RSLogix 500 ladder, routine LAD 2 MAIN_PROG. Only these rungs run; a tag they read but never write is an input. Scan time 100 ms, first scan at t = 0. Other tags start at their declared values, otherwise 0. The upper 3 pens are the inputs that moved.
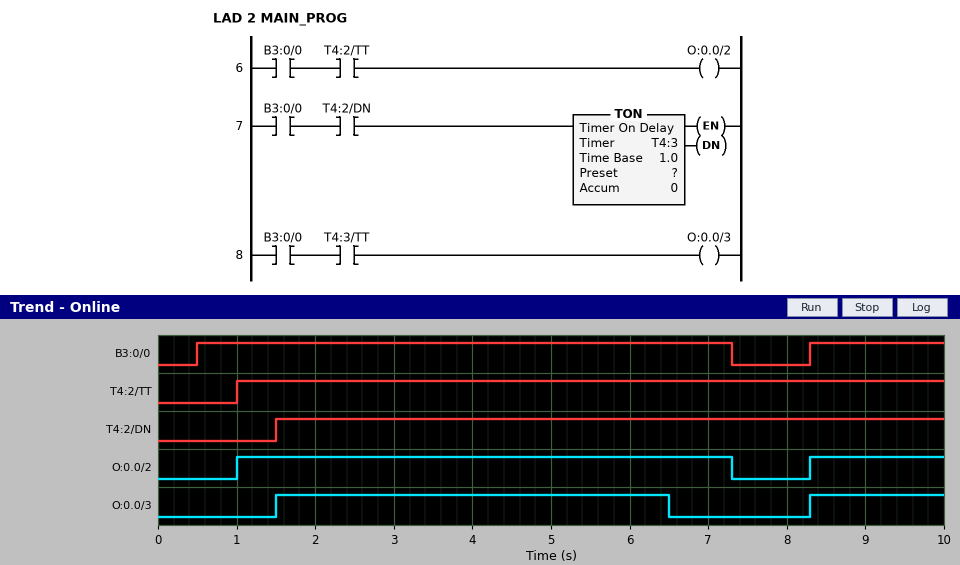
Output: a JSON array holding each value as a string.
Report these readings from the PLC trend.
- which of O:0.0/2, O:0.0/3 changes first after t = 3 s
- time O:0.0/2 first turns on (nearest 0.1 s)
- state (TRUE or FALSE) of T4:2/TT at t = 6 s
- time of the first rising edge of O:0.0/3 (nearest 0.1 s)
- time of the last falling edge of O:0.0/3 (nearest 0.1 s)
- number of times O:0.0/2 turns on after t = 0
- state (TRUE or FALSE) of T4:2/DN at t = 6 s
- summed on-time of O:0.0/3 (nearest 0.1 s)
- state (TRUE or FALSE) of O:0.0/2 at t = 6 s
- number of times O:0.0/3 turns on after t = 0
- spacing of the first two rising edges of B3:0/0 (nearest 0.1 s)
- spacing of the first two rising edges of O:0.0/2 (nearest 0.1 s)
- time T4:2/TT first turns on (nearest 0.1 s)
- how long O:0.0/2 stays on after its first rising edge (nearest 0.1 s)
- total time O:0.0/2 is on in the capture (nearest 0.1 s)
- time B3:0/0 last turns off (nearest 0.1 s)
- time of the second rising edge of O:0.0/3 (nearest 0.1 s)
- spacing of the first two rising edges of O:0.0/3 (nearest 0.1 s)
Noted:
["O:0.0/3", "1.0 s", "TRUE", "1.5 s", "6.5 s", "2", "TRUE", "6.7 s", "TRUE", "2", "7.8 s", "7.3 s", "1.0 s", "6.3 s", "8.0 s", "7.3 s", "8.3 s", "6.8 s"]
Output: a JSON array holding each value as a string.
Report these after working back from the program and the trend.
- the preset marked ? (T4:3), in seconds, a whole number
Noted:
["5 s"]
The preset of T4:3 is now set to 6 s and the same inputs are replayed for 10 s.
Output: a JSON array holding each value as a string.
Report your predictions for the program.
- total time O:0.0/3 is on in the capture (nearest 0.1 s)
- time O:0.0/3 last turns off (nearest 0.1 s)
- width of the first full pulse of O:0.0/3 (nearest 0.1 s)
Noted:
["7.5 s", "7.3 s", "5.8 s"]
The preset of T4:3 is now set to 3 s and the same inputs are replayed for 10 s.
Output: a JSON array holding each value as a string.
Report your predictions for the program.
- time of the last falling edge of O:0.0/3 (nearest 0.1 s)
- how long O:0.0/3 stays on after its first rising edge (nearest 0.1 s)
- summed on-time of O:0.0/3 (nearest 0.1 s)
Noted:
["4.5 s", "3.0 s", "4.7 s"]
